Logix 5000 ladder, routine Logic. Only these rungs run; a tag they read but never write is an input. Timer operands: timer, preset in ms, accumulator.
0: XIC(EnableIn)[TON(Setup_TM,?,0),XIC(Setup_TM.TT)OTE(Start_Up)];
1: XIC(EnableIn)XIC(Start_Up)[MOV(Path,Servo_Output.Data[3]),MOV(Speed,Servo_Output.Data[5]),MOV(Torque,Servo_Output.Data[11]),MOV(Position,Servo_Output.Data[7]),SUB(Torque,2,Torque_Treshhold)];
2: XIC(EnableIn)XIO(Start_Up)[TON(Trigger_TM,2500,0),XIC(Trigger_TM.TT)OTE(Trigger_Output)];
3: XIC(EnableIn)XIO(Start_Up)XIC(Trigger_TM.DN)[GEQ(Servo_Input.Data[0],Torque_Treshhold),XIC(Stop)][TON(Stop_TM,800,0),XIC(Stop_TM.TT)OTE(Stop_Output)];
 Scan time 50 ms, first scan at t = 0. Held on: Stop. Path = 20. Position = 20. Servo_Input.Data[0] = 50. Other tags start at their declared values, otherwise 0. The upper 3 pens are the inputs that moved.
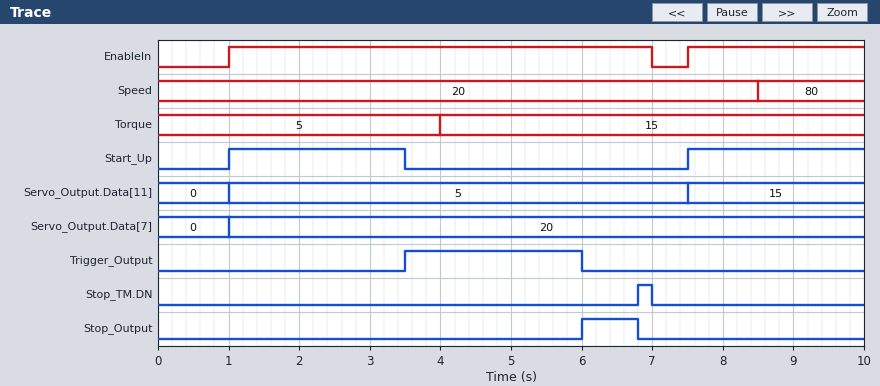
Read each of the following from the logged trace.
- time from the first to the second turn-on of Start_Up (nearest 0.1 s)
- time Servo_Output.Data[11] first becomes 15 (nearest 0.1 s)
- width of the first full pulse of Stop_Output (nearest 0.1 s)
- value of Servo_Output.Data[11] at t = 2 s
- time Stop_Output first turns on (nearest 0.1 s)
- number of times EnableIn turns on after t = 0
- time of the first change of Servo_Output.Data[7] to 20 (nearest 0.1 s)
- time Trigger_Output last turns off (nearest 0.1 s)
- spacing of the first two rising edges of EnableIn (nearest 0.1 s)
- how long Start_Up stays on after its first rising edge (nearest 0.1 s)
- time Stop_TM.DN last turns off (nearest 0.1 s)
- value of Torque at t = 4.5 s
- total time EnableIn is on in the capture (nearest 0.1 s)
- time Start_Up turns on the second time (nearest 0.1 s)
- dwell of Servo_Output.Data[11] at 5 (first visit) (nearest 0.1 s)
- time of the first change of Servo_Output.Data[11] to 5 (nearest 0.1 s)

6.5 s
7.5 s
0.8 s
5
6.0 s
2
1.0 s
6.0 s
6.5 s
2.5 s
7.0 s
15
8.5 s
7.5 s
6.5 s
1.0 s
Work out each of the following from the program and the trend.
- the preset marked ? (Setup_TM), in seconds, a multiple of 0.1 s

2.5 s
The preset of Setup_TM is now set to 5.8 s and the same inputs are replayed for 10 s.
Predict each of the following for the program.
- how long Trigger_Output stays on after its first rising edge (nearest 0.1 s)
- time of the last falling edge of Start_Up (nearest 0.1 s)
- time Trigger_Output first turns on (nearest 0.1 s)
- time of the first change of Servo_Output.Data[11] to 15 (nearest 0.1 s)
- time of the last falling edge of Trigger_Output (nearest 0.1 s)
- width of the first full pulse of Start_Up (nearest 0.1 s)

0.2 s
6.8 s
6.8 s
4.0 s
7.0 s
5.8 s
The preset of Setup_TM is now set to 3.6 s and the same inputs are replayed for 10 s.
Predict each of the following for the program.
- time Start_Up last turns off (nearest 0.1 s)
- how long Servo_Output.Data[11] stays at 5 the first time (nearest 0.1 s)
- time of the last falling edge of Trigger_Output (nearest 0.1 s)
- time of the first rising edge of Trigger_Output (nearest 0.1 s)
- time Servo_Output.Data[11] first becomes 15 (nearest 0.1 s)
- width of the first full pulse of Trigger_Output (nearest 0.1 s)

4.6 s
3.0 s
7.0 s
4.6 s
4.0 s
2.4 s
